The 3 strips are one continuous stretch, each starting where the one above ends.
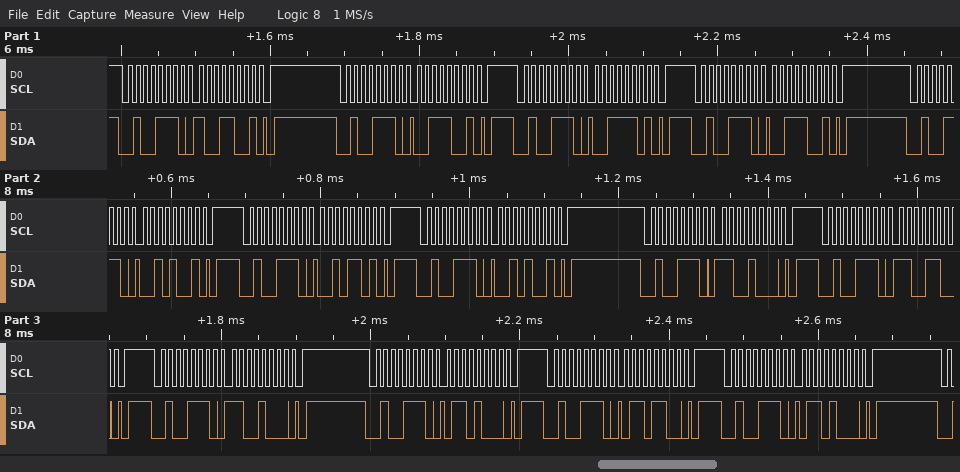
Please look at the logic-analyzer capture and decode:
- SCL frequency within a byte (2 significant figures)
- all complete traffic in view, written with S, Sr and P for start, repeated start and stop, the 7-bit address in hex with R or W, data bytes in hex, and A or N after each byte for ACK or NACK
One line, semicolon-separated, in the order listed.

100 kHz; S 27W A 99 A P S 27W A 39 A P S 27W A 3D A P S 27W A 39 A P S 27W A 29 A P S 27W A 2D A P S 27W A 29 A P S 27W A C8 A P S 27W A CC A P S 27W A C8 A P S 27W A 68 A P S 27W A 6C A P S 27W A 68 A P
